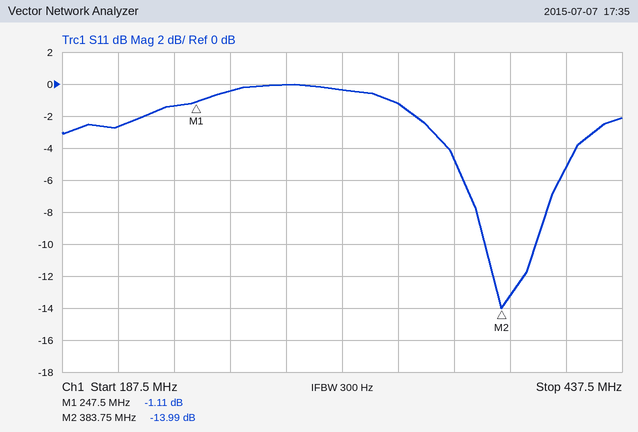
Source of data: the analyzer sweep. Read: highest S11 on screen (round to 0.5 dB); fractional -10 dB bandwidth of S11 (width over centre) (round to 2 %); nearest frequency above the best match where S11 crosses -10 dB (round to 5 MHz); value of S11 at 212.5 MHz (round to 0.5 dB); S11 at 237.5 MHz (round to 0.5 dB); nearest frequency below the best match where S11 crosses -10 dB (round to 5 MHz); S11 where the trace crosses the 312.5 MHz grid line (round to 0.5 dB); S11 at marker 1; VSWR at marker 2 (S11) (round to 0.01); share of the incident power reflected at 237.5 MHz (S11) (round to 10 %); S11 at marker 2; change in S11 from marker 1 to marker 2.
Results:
0.0 dB
6 %
400 MHz
-2.5 dB
-1.5 dB
375 MHz
-0.5 dB
-1.11 dB
1.50
70 %
-13.99 dB
-12.88 dB
